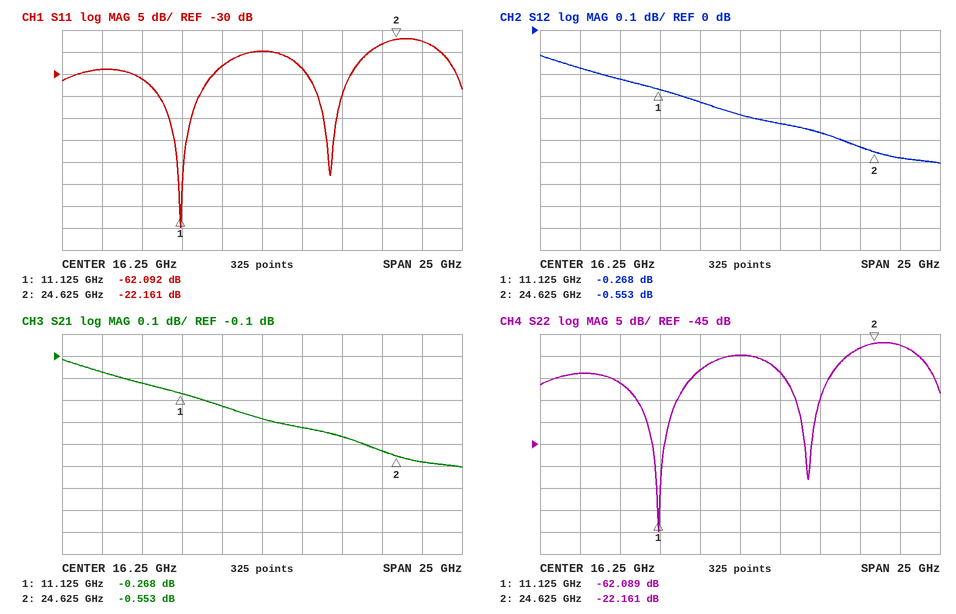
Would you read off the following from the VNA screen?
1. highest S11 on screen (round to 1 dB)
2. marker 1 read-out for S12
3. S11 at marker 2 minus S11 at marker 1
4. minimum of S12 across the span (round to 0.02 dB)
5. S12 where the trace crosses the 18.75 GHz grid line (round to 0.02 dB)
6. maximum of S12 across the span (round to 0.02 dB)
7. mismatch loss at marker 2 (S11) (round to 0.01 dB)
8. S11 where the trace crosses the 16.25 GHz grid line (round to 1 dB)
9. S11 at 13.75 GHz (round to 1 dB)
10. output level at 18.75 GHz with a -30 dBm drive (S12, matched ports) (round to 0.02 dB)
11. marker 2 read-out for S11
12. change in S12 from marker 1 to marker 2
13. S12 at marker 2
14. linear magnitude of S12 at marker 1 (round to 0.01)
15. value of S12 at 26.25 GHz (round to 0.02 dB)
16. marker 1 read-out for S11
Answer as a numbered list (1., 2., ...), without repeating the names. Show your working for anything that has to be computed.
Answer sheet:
1. -22 dB
2. -0.268 dB
3. -22.161 − (-62.092) = 39.931 dB
4. -0.60 dB
5. -0.42 dB
6. -0.12 dB
7. −10 log10(1 − 10^(-22.161/10)) ≈ 0.03 dB
8. -25 dB
9. -28 dB
10. -30 dBm + (-0.42 dB) = -30.42 dBm
11. -22.161 dB
12. -0.553 − (-0.268) = -0.285 dB
13. -0.553 dB
14. 10^(-0.268/20) ≈ 0.97
15. -0.58 dB
16. -62.092 dB
